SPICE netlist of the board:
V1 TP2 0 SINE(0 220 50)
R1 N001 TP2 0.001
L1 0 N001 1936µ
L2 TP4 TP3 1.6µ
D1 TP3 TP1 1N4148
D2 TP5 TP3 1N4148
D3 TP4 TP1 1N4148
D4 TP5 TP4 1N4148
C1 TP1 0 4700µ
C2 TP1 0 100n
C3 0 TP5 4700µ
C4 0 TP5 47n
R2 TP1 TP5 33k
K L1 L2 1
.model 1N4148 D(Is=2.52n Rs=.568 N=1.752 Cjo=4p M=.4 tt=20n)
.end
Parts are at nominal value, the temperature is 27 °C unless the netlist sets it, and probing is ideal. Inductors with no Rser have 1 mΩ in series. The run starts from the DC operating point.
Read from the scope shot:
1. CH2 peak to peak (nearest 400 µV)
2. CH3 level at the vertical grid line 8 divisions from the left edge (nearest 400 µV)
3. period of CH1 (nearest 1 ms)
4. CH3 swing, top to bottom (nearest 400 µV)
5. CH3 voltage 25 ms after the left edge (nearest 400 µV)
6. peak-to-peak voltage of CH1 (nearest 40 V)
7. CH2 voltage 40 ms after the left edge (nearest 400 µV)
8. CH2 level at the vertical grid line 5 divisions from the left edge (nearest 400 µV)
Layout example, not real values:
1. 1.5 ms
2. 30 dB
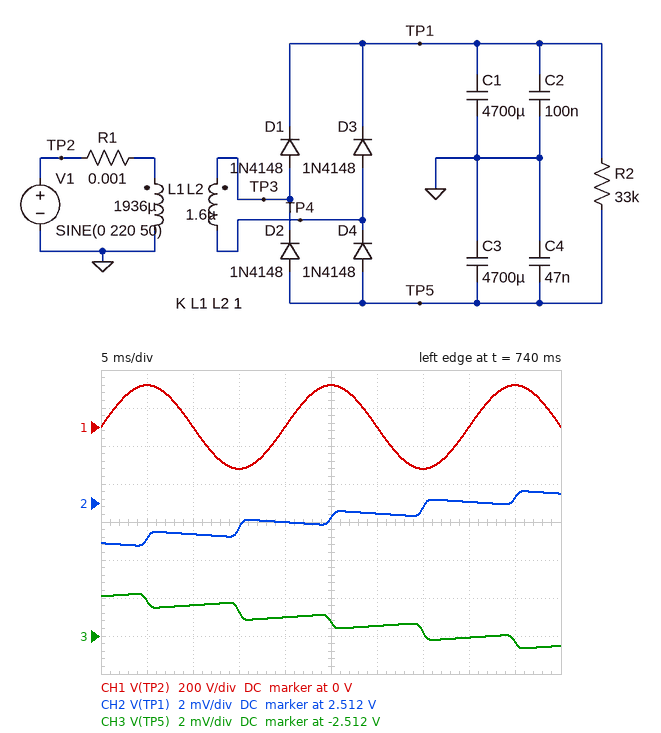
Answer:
1. 2.8 mV
2. -2.5120 V
3. 20 ms
4. 2.8 mV
5. -2.5112 V
6. 440 V
7. 2.5120 V
8. 2.5112 V
